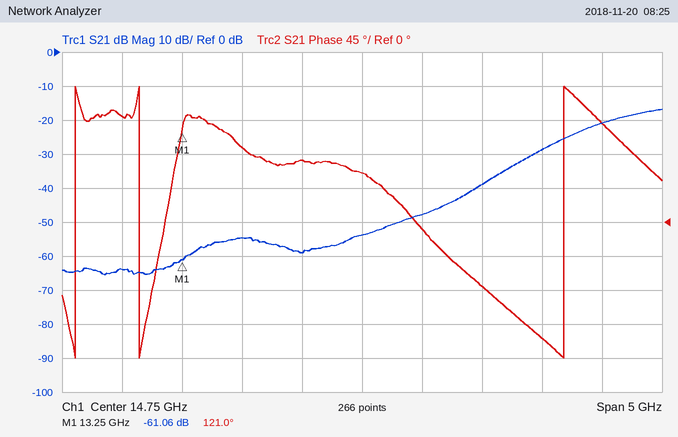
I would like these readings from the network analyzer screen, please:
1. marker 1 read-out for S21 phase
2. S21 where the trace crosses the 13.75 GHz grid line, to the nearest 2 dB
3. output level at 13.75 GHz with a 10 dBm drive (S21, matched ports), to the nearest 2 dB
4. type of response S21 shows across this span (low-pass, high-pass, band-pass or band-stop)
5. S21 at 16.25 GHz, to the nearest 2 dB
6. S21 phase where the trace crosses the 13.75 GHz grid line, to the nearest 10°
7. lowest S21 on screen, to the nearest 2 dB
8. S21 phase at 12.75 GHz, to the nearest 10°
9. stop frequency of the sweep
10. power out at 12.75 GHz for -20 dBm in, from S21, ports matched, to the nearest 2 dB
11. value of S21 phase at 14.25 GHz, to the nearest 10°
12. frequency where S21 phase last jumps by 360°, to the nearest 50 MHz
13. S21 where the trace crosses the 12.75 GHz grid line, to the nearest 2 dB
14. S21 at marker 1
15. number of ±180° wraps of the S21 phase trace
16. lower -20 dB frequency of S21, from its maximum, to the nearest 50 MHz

121.0°
-54 dB
-44 dBm
high-pass
-28 dB
100°
-66 dB
140°
17.25 GHz
-84 dBm
80°
16.45 GHz
-64 dB
-61.06 dB
3
15.85 GHz
